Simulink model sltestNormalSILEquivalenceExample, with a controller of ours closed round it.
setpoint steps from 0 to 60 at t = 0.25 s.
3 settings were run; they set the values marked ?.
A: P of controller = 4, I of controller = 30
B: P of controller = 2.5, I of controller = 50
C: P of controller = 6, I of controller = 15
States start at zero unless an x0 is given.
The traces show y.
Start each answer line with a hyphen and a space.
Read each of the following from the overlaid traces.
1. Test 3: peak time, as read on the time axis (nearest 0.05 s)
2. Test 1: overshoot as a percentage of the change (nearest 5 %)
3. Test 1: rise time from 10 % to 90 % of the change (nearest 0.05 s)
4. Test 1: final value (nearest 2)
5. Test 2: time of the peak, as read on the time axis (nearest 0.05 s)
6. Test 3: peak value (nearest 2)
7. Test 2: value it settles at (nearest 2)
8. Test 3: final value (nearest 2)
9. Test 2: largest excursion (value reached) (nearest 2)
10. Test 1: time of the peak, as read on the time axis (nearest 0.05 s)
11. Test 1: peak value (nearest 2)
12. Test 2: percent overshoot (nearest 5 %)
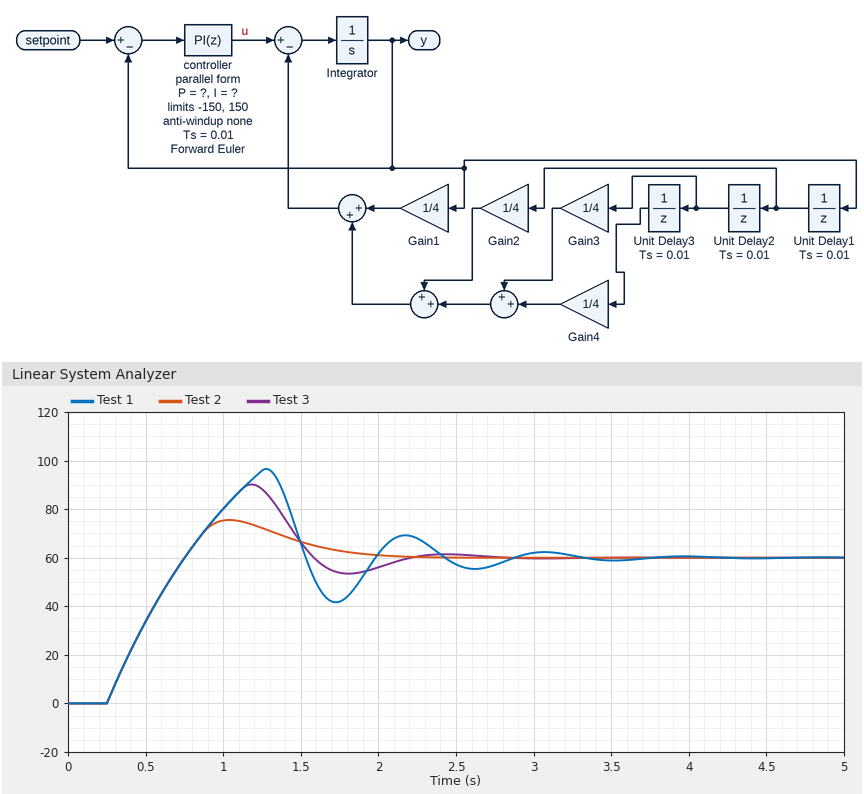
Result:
- 1.20 s
- 60 %
- 0.40 s
- 60
- 1.05 s
- 90
- 60
- 60
- 76
- 1.30 s
- 96
- 25 %
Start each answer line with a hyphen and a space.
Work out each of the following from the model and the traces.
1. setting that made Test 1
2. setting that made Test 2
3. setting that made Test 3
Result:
- B
- C
- A
